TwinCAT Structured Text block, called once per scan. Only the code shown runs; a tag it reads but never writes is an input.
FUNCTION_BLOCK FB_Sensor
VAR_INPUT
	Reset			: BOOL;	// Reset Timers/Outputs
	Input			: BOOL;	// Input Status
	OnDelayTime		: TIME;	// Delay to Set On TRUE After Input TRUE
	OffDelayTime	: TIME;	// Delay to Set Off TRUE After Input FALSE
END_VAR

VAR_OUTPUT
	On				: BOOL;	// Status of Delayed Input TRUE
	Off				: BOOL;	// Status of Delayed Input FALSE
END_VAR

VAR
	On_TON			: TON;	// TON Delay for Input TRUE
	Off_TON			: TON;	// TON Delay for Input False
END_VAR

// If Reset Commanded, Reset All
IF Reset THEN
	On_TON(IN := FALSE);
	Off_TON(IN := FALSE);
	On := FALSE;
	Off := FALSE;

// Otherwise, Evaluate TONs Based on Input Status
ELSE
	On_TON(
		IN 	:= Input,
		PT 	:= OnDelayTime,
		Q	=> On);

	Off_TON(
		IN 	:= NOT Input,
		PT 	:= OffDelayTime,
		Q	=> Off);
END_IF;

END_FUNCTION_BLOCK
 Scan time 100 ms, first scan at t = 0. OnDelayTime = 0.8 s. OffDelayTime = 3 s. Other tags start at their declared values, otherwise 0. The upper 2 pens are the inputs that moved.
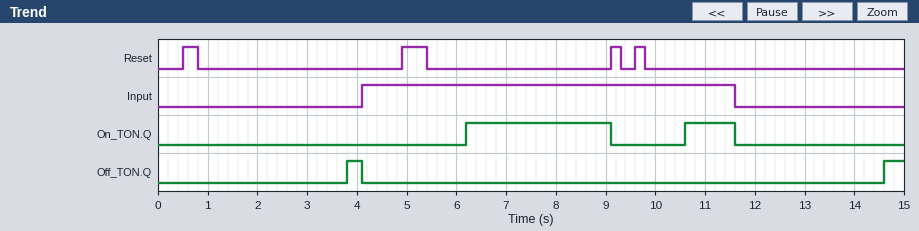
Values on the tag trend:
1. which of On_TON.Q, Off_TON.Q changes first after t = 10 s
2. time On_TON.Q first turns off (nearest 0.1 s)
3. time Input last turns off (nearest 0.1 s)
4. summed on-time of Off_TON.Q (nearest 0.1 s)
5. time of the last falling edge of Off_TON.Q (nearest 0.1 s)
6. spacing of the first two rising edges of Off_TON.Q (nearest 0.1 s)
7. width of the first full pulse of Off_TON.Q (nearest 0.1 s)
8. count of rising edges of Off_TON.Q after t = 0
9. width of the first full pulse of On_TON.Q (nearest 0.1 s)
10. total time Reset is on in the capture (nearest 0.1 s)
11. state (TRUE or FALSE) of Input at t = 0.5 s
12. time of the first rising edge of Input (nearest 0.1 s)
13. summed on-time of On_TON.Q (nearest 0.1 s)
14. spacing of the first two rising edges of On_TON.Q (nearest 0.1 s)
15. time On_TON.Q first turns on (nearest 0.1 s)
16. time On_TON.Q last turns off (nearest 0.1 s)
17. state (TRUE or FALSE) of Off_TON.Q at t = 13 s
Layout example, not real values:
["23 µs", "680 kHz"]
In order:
["On_TON.Q", "9.1 s", "11.6 s", "0.7 s", "4.1 s", "10.8 s", "0.3 s", "2", "2.9 s", "1.2 s", "FALSE", "4.1 s", "3.9 s", "4.4 s", "6.2 s", "11.6 s", "FALSE"]
